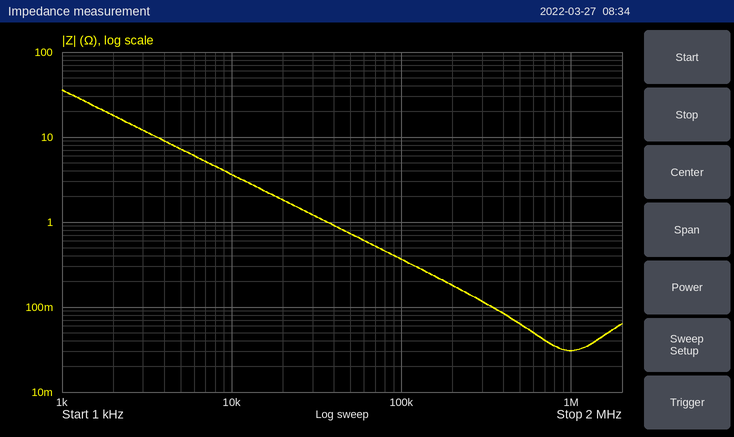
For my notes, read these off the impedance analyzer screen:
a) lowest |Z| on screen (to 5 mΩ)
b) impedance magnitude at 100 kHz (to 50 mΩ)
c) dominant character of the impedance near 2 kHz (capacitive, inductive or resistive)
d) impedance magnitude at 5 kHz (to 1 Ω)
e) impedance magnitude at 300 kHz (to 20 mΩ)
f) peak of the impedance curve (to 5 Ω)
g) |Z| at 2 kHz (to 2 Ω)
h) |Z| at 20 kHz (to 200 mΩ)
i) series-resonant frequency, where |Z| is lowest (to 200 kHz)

30 mΩ
350 mΩ
capacitive
7 Ω
120 mΩ
35 Ω
18 Ω
1.8 Ω
1.0 MHz
